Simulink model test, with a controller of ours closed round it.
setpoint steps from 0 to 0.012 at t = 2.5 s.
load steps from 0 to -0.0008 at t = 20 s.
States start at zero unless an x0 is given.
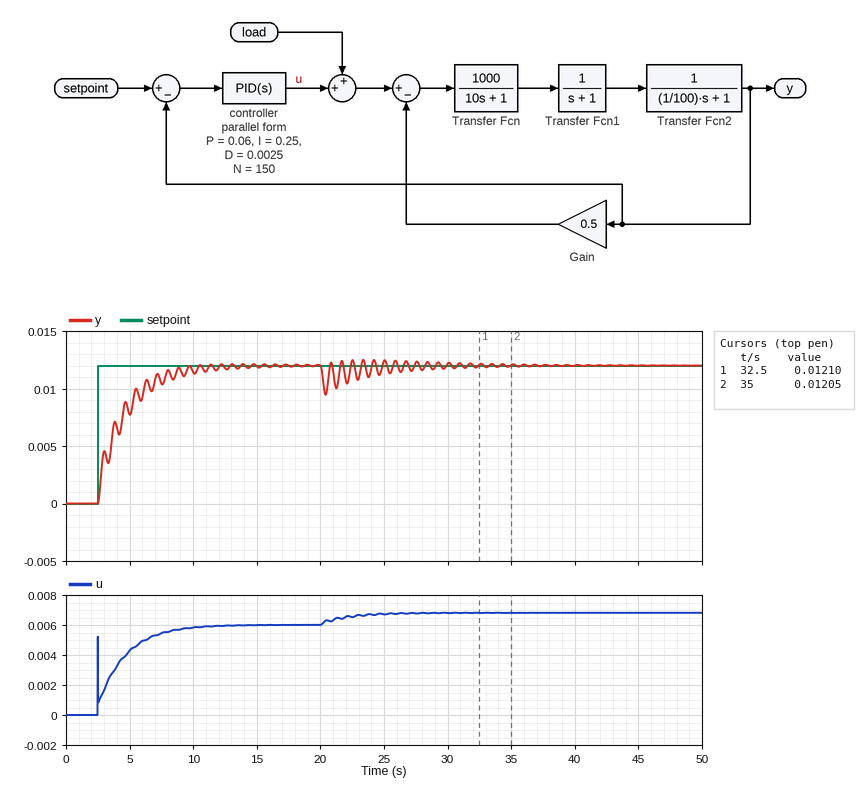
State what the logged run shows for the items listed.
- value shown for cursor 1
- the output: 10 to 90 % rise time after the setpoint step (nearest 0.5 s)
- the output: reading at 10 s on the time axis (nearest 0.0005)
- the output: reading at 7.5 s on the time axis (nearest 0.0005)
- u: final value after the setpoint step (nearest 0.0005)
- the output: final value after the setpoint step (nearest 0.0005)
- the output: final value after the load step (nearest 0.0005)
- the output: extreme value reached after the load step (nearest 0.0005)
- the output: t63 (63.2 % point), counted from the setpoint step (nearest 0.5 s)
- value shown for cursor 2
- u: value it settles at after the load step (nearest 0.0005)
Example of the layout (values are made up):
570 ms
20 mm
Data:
0.01210
4.5 s
0.0115
0.0105
0.0060
0.0120
0.0120
0.0095
2.0 s
0.01205
0.0070
